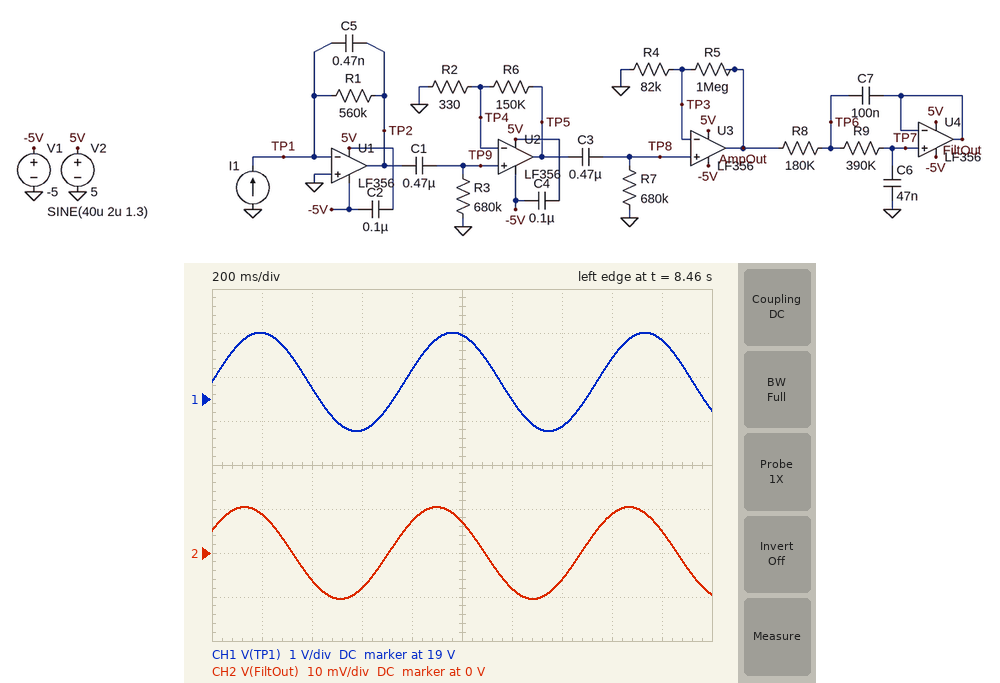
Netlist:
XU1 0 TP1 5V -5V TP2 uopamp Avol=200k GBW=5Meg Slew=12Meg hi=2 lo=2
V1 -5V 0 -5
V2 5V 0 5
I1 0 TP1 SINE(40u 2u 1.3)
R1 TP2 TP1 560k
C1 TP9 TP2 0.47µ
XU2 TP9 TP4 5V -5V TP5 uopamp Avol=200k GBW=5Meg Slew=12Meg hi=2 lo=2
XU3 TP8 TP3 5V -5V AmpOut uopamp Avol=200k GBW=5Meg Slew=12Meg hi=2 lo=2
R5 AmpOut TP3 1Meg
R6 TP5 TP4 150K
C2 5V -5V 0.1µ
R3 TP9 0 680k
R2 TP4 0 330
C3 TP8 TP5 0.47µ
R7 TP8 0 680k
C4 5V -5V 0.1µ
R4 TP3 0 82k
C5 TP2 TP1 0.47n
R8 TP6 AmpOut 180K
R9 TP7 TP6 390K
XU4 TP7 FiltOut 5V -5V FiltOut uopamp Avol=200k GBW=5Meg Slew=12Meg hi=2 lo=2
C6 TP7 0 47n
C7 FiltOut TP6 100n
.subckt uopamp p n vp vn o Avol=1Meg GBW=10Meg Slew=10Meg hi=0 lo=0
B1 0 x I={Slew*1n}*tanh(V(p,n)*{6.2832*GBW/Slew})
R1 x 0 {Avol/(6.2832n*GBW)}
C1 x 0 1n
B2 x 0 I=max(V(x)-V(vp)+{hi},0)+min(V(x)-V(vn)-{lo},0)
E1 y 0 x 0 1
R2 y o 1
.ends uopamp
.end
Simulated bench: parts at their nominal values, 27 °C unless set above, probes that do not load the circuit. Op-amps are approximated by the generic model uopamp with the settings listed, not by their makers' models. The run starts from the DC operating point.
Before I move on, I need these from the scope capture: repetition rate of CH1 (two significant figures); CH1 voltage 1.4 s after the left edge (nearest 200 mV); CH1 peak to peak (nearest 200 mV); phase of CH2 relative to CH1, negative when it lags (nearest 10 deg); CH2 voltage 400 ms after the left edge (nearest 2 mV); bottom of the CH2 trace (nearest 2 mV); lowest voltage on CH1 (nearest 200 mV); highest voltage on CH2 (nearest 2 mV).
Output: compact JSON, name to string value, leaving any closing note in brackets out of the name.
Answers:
{"repetition rate of CH1": "1.3 Hz", "CH1 voltage 1.4 s after the left edge": "18.4 V", "CH1 peak to peak": "2.2 V", "phase of CH2 relative to CH1, negative when it lags": "30 deg", "CH2 voltage 400 ms after the left edge": "-6 mV", "bottom of the CH2 trace": "-10 mV", "lowest voltage on CH1": "18.2 V", "highest voltage on CH2": "10 mV"}
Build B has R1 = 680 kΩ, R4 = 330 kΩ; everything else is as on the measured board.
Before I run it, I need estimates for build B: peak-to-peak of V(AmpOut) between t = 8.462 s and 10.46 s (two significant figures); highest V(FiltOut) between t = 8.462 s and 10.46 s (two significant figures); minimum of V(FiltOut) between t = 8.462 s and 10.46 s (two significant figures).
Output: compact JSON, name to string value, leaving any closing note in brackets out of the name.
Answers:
{"peak-to-peak of V(AmpOut) between t = 8.462 s and 10.46 s": "6.4 mV", "highest V(FiltOut) between t = 8.462 s and 10.46 s": "3.2 mV", "minimum of V(FiltOut) between t = 8.462 s and 10.46 s": "-3.2 mV"}
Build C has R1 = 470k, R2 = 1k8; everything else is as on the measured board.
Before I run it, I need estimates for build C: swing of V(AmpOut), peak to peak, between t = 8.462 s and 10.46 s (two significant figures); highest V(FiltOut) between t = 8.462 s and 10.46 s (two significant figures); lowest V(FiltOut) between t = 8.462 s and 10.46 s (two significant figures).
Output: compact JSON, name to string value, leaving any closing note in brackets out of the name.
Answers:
{"swing of V(AmpOut), peak to peak, between t = 8.462 s and 10.46 s": "3.9 mV", "highest V(FiltOut) between t = 8.462 s and 10.46 s": "1.9 mV", "lowest V(FiltOut) between t = 8.462 s and 10.46 s": "-1.9 mV"}
